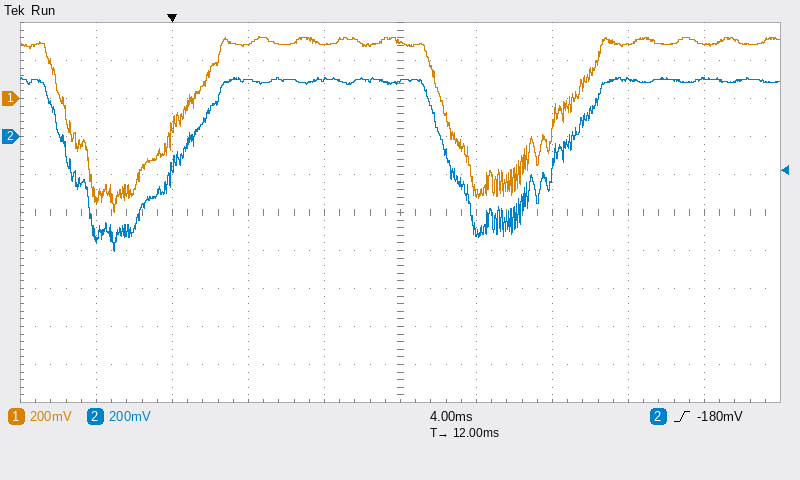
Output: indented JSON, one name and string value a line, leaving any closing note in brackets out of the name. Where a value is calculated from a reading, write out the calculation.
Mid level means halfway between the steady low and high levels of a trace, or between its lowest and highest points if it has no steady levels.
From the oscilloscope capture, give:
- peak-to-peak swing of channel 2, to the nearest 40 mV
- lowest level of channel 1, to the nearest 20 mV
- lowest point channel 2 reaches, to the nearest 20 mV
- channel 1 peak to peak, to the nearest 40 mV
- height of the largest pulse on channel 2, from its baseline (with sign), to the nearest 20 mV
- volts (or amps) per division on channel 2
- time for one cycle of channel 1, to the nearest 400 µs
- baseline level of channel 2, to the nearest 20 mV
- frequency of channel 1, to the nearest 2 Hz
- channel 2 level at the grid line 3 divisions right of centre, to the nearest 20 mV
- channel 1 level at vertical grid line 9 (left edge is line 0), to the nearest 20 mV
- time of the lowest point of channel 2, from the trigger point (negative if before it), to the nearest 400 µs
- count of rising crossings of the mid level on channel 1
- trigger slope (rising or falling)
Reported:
{
  "peak-to-peak swing of channel 2, to the nearest 40 mV": "920 mV",
  "lowest level of channel 1, to the nearest 20 mV": "-600 mV",
  "lowest point channel 2 reaches, to the nearest 20 mV": "-600 mV",
  "channel 1 peak to peak, to the nearest 40 mV": "920 mV",
  "height of the largest pulse on channel 2, from its baseline (with sign), to the nearest 20 mV": "-600 mV − (300 mV) = -900 mV",
  "volts (or amps) per division on channel 2": "200 mV",
  "time for one cycle of channel 1, to the nearest 400 µs": "20.0 ms",
  "baseline level of channel 2, to the nearest 20 mV": "300 mV",
  "frequency of channel 1, to the nearest 2 Hz": "1 / 20.0 ms ≈ 50 Hz",
  "channel 2 level at the grid line 3 divisions right of centre, to the nearest 20 mV": "300 mV",
  "channel 1 level at vertical grid line 9 (left edge is line 0), to the nearest 20 mV": "280 mV",
  "time of the lowest point of channel 2, from the trigger point (negative if before it), to the nearest 400 µs": "-3.2 ms",
  "count of rising crossings of the mid level on channel 1": "2",
  "trigger slope": "rising"
}
